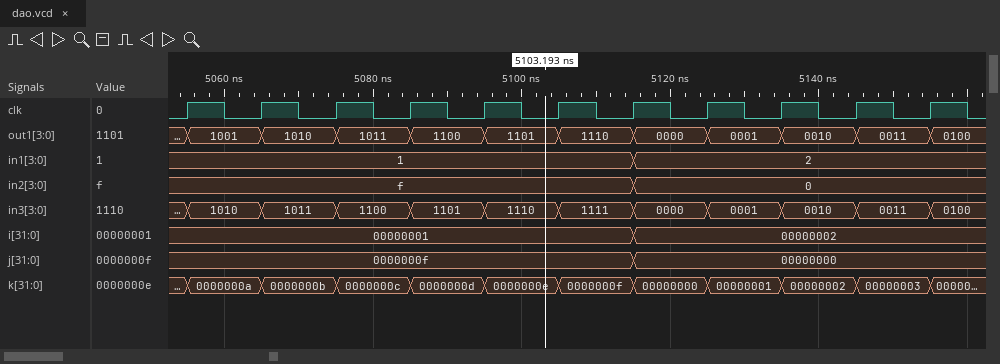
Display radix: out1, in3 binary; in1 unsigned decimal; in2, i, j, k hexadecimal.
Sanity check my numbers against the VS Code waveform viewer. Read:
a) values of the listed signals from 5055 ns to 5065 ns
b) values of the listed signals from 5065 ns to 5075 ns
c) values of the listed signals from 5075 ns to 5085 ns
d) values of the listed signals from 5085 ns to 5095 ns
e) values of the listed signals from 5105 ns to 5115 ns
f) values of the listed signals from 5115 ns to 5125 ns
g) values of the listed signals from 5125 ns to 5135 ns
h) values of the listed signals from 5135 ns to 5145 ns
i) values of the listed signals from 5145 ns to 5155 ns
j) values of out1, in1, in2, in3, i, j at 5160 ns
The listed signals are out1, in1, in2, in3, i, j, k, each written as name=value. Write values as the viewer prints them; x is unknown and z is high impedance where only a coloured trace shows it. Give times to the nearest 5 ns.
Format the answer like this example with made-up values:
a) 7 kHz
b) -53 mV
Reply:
a) out1=1001, in1=1, in2=f, in3=1010, i=00000001, j=0000000f, k=0000000a
b) out1=1010, in1=1, in2=f, in3=1011, i=00000001, j=0000000f, k=0000000b
c) out1=1011, in1=1, in2=f, in3=1100, i=00000001, j=0000000f, k=0000000c
d) out1=1100, in1=1, in2=f, in3=1101, i=00000001, j=0000000f, k=0000000d
e) out1=1110, in1=1, in2=f, in3=1111, i=00000001, j=0000000f, k=0000000f
f) out1=0000, in1=2, in2=0, in3=0000, i=00000002, j=00000000, k=00000000
g) out1=0001, in1=2, in2=0, in3=0001, i=00000002, j=00000000, k=00000001
h) out1=0010, in1=2, in2=0, in3=0010, i=00000002, j=00000000, k=00000002
i) out1=0011, in1=2, in2=0, in3=0011, i=00000002, j=00000000, k=00000003
j) out1=0100, in1=2, in2=0, in3=0100, i=00000002, j=00000000
